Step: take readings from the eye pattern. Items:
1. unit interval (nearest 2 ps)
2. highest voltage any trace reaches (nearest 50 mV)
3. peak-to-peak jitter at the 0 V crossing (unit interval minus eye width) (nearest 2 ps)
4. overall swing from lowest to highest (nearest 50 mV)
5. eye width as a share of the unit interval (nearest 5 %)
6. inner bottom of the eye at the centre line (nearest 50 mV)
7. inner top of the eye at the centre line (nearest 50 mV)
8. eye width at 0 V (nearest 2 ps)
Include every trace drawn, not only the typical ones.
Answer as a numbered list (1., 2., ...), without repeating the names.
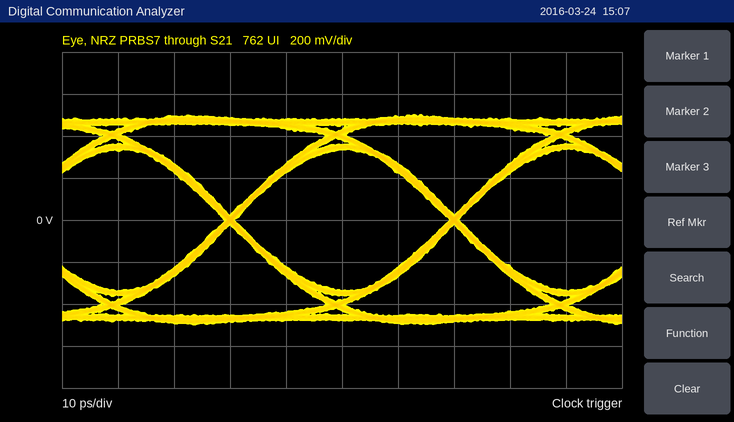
1. 40 ps
2. 500 mV
3. 2 ps
4. 1.00 V
5. 95 %
6. -350 mV
7. 350 mV
8. 38 ps
